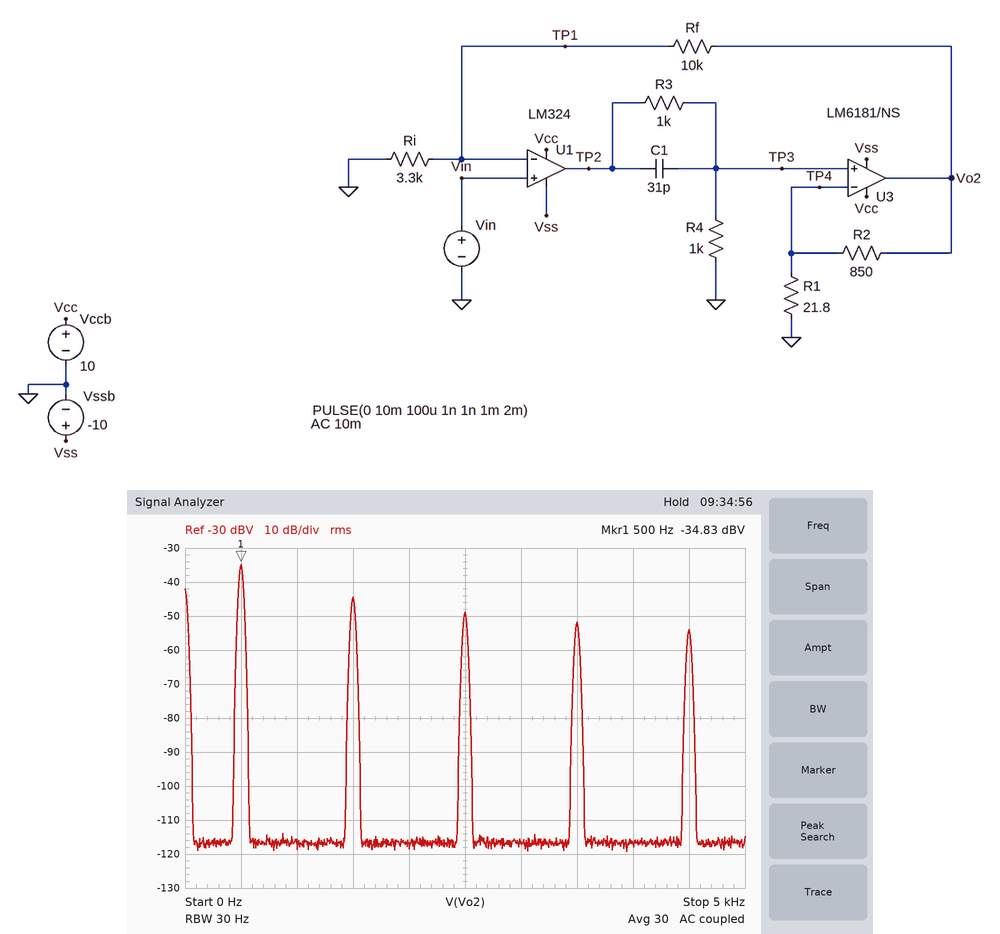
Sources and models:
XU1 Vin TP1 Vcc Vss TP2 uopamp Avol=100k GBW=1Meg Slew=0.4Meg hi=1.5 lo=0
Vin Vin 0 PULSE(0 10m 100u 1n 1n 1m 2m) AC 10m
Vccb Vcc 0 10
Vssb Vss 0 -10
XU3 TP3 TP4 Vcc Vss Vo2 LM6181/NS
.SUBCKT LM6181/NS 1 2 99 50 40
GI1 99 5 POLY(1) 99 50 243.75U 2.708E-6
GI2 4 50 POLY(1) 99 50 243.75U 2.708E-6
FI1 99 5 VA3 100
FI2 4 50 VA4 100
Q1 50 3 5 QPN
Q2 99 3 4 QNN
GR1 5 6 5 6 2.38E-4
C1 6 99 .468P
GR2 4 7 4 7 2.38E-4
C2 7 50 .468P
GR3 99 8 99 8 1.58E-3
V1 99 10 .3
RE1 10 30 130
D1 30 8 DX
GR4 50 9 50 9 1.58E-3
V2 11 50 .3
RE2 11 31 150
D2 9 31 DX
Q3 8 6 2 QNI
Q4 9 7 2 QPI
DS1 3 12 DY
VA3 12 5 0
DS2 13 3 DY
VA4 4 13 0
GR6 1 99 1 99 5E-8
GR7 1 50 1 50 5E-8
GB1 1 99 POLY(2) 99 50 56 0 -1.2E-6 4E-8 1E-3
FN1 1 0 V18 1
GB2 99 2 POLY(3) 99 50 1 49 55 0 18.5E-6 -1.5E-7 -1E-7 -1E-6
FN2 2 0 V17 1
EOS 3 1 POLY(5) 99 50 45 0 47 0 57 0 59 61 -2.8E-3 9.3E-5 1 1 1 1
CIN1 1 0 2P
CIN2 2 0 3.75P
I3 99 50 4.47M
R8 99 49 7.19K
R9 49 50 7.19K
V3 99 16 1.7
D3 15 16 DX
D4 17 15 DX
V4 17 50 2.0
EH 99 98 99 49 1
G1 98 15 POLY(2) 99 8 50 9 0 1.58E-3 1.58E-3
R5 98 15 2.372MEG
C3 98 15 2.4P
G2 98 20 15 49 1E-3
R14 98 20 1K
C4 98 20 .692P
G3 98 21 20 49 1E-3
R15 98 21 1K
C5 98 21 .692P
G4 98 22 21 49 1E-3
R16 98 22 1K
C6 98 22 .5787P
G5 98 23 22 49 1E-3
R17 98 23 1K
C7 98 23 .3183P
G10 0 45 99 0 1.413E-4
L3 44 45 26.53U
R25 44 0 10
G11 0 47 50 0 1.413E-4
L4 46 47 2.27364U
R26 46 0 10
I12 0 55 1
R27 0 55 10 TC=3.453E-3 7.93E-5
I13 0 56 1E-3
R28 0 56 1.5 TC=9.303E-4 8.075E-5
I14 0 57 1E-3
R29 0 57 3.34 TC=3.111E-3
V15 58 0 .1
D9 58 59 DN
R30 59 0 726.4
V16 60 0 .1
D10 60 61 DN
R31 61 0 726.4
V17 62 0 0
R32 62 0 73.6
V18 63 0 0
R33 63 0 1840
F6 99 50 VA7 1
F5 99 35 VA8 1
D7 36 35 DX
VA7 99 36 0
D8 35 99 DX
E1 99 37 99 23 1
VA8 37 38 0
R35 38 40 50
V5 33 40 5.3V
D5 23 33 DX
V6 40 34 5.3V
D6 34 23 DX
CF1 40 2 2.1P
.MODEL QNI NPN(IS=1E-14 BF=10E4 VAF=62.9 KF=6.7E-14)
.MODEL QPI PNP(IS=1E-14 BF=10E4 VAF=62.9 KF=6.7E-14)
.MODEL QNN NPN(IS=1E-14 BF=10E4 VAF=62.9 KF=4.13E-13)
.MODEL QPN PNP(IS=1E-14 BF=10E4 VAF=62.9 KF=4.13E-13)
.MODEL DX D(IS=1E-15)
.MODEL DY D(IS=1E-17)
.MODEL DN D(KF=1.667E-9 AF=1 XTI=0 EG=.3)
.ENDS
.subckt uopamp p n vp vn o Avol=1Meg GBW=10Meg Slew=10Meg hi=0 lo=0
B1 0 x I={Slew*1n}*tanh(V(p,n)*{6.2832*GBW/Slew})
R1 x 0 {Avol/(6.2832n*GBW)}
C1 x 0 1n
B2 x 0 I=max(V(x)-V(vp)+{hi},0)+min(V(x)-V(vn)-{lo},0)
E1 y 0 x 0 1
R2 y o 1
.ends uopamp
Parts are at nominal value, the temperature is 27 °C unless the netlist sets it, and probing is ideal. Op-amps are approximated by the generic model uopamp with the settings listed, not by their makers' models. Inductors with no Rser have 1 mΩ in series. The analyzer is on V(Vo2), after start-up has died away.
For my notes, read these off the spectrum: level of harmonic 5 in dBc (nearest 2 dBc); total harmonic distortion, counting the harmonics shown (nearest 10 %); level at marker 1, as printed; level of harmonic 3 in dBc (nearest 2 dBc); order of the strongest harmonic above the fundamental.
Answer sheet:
-14 dBc
40 %
-34.83 dBV
-10 dBc
3
